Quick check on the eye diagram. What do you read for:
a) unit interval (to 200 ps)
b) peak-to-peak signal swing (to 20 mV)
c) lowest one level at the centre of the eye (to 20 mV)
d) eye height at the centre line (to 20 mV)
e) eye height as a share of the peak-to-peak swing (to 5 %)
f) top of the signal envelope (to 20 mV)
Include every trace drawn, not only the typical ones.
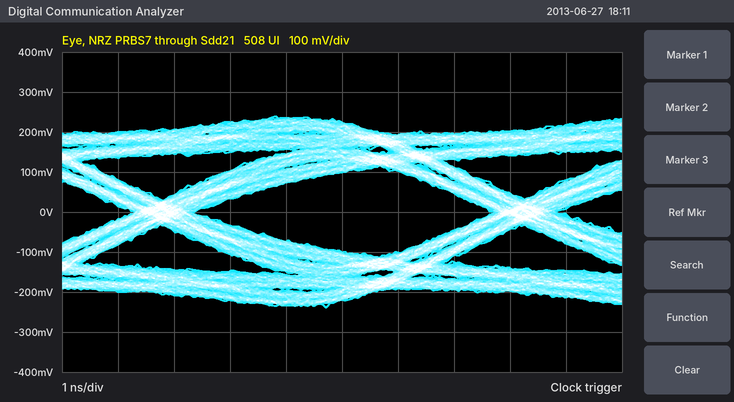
6.4 ns
480 mV
100 mV
200 mV
40 %
240 mV
